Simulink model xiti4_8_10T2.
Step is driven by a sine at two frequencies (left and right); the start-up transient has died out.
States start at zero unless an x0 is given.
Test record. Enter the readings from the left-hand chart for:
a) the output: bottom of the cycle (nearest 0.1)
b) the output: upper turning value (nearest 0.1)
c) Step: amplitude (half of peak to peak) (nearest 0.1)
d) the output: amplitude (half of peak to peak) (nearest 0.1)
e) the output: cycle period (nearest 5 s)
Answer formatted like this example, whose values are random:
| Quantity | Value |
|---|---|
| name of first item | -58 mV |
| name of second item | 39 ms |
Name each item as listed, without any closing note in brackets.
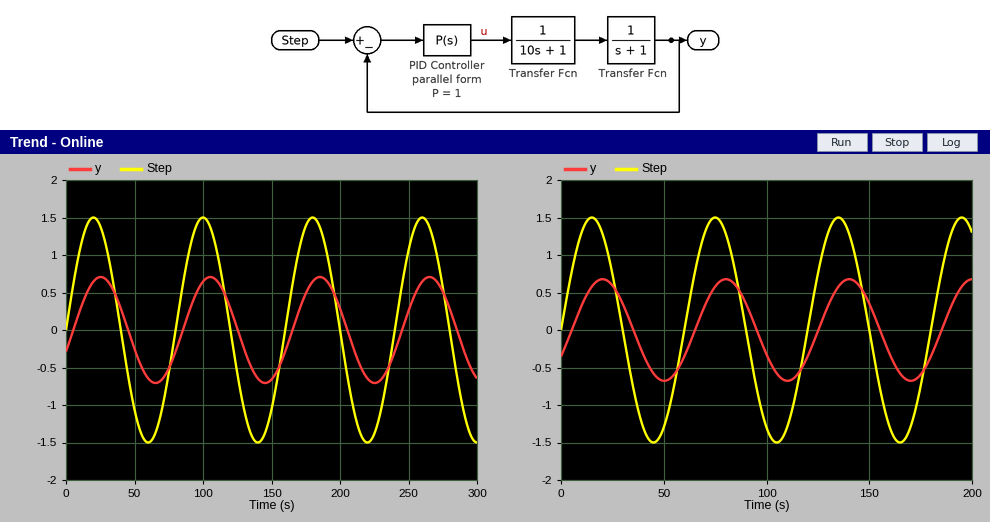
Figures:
| Quantity | Value |
|---|---|
| the output: bottom of the cycle | -0.7 |
| the output: upper turning value | 0.7 |
| Step: amplitude (half of peak to peak) | 1.5 |
| the output: amplitude (half of peak to peak) | 0.7 |
| the output: cycle period | 80 s |
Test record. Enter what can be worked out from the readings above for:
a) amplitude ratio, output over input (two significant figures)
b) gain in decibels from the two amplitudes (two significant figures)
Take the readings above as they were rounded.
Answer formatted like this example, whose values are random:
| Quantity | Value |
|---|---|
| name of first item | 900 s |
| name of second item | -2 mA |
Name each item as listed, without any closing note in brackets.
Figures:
| Quantity | Value |
|---|---|
| amplitude ratio, output over input | 0.47 |
| gain in decibels from the two amplitudes | -6.6 dB |
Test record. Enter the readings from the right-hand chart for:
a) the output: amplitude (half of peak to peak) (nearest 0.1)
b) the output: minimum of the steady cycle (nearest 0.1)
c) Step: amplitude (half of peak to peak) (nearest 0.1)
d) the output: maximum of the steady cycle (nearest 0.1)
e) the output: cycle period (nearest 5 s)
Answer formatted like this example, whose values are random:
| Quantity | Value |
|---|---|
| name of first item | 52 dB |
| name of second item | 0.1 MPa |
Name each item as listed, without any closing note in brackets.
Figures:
| Quantity | Value |
|---|---|
| the output: amplitude (half of peak to peak) | 0.7 |
| the output: minimum of the steady cycle | -0.7 |
| Step: amplitude (half of peak to peak) | 1.5 |
| the output: maximum of the steady cycle | 0.7 |
| the output: cycle period | 60 s |
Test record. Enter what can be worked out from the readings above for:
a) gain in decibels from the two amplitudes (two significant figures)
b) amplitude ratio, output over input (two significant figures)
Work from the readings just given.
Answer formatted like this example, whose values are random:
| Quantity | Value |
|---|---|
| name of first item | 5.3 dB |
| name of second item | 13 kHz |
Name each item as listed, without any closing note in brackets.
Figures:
| Quantity | Value |
|---|---|
| gain in decibels from the two amplitudes | -6.6 dB |
| amplitude ratio, output over input | 0.47 |
